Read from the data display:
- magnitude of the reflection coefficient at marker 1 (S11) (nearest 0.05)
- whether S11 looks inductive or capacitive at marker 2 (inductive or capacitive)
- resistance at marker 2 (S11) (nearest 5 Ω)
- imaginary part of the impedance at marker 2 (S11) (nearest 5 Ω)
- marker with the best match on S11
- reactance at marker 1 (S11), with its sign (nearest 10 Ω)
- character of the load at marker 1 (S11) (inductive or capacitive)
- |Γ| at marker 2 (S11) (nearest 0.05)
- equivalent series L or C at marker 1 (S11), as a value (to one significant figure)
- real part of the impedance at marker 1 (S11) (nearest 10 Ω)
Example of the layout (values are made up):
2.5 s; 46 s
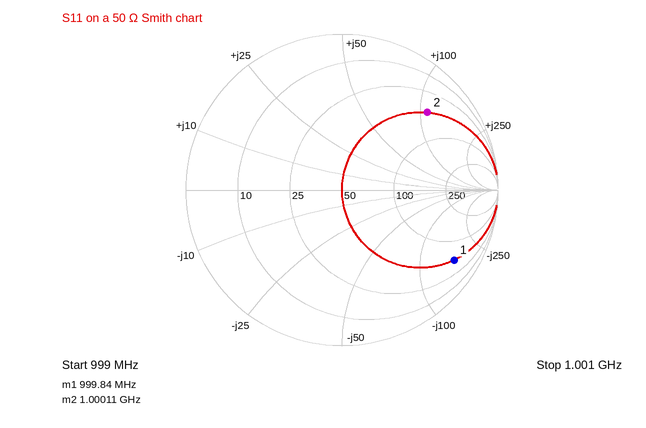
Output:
0.85; inductive; 50 Ω; +110 Ω; marker 2; -160 Ω; capacitive; 0.75; 1.0 pF; 50 Ω
